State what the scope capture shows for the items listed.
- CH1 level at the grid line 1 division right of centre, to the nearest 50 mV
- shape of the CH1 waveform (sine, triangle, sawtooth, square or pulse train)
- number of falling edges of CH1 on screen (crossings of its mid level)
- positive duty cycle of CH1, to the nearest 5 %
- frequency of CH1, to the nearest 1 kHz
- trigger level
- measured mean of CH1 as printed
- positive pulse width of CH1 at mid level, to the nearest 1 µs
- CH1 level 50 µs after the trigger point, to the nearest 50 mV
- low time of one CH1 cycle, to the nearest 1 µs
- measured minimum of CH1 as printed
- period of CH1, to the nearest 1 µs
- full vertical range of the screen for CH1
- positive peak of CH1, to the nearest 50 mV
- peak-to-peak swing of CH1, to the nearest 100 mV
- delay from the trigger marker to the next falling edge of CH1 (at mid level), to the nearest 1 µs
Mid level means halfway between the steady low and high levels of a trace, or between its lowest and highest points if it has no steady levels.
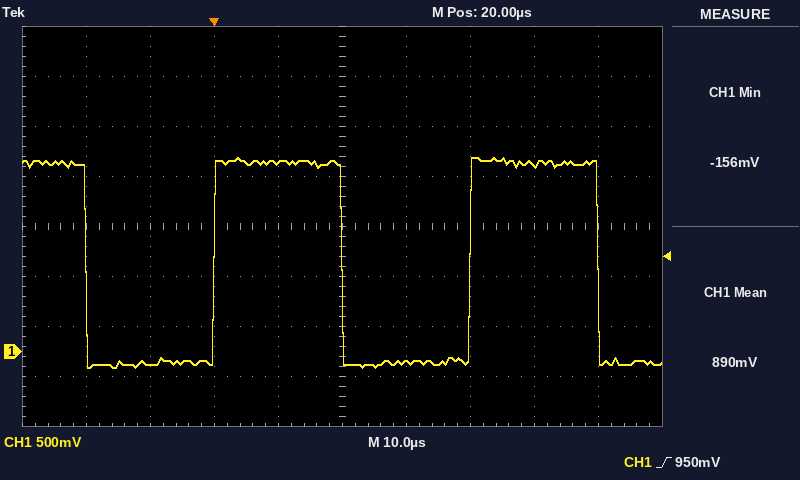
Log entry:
-100 mV
square
3
50 %
25 kHz
950 mV
890 mV
20 µs
1.85 V
20 µs
-156 mV
40 µs
4 V
1.95 V
2.10 V
20 µs
